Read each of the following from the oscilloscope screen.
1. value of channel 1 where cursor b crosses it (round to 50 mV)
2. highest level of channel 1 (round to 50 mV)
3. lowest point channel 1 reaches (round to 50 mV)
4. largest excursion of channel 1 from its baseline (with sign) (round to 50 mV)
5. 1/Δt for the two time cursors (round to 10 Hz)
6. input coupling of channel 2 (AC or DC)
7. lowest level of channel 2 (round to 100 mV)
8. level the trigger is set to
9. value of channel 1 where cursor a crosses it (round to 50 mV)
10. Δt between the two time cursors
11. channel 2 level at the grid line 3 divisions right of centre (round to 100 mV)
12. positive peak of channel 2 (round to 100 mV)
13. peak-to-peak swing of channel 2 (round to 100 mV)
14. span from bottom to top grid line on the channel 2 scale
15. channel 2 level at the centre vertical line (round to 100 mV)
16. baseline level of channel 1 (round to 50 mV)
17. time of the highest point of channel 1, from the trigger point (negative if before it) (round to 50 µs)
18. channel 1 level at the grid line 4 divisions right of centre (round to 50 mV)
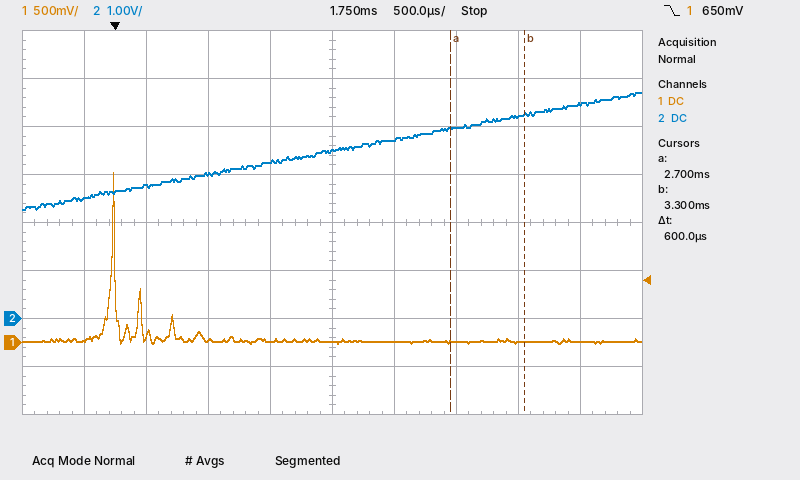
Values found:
0 mV
1.75 V
0 mV
+1.75 V
1.67 kHz
DC
2.3 V
650 mV
0 mV
600 µs
4.2 V
4.7 V
2.4 V
8 V
3.5 V
0 mV
0 µs
0 mV
